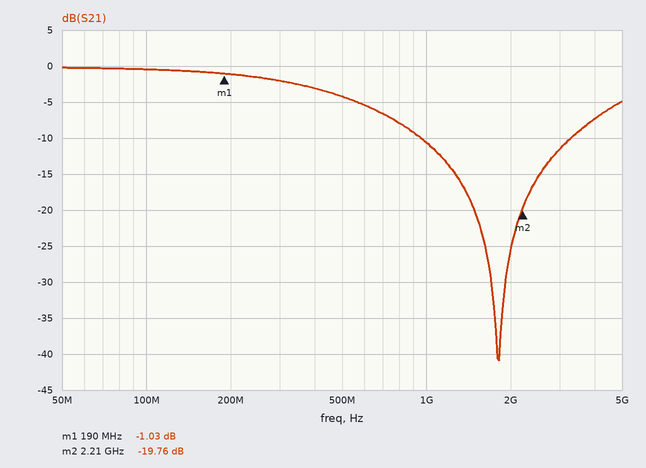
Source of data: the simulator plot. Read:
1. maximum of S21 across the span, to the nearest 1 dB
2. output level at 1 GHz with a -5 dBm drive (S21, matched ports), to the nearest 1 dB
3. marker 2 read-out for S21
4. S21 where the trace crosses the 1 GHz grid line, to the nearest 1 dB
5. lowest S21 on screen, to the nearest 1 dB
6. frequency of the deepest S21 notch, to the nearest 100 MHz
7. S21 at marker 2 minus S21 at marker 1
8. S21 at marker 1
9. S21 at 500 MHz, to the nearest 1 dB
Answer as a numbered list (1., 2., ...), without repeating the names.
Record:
1. 0 dB
2. -16 dBm
3. -19.76 dB
4. -11 dB
5. -41 dB
6. 1.8 GHz
7. -18.73 dB
8. -1.03 dB
9. -4 dB
